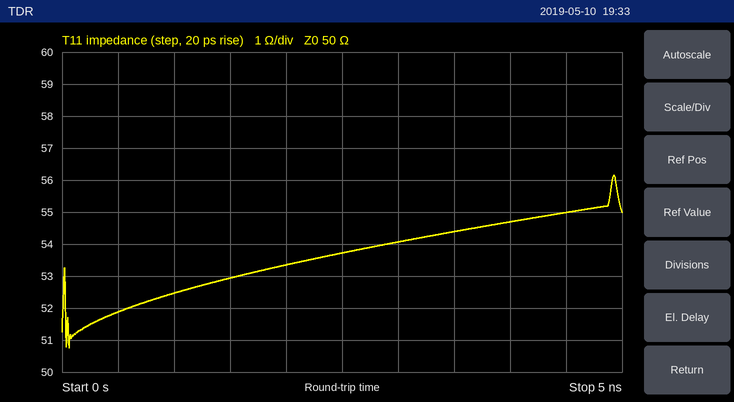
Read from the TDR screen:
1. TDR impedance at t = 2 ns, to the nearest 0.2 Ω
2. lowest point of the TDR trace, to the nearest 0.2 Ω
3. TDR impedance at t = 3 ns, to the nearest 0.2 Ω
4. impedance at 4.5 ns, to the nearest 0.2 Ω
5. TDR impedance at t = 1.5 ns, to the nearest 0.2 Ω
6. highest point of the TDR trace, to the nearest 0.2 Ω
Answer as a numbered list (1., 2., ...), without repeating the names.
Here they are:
1. 53.4 Ω
2. 50.8 Ω
3. 54.0 Ω
4. 55.0 Ω
5. 53.0 Ω
6. 56.2 Ω
